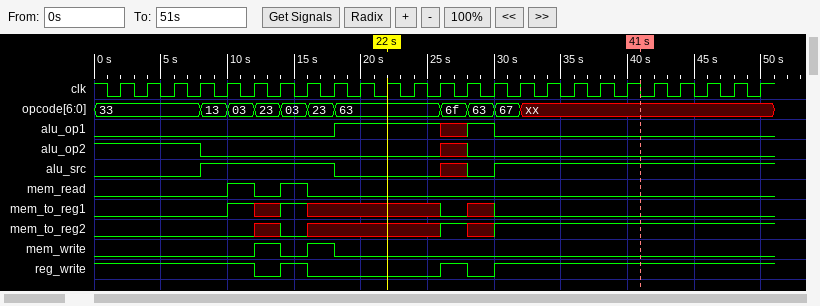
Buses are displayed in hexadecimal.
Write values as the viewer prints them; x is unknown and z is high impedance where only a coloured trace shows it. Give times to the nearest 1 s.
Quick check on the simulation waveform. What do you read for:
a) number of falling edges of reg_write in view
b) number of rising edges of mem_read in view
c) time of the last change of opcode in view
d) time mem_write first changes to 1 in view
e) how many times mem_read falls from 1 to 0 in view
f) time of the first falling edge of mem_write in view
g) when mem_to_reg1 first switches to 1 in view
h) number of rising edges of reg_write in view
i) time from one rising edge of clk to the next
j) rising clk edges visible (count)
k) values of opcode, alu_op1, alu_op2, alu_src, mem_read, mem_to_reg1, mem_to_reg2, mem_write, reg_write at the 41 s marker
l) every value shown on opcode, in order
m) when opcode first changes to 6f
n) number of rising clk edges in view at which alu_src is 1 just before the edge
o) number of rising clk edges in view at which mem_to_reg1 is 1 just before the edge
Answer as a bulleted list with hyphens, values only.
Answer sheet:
- 3
- 2
- 32 s
- 12 s
- 2
- 14 s
- 10 s
- 3
- 2 s
- 25
- opcode=xx, alu_op1=0, alu_op2=0, alu_src=1, mem_read=0, mem_to_reg1=0, mem_to_reg2=1, mem_write=0, reg_write=1
- 33, 13, 03, 23, 03, 23, 63, 6f, 63, 67, xx
- 26 s
- 15
- 2
